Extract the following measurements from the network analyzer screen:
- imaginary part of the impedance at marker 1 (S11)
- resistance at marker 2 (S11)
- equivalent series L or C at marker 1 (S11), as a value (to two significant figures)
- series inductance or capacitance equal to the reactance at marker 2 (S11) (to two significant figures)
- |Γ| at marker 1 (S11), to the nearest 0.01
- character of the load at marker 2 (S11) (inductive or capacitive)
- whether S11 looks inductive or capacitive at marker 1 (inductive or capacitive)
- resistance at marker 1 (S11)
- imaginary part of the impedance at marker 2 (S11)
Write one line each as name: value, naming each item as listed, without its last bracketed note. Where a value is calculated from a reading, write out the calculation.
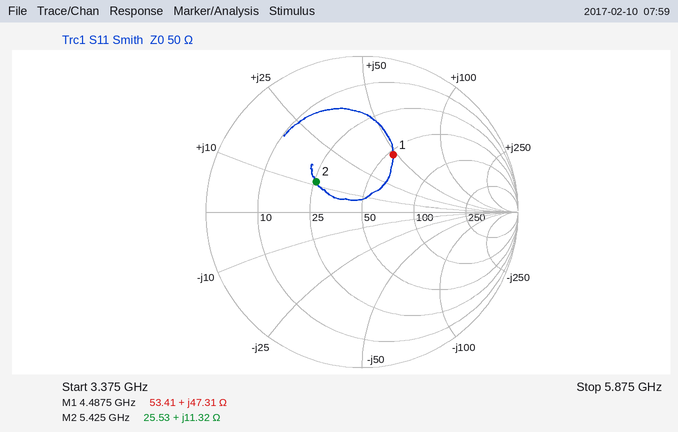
imaginary part of the impedance at marker 1: +47.31 Ω
resistance at marker 2: 25.53 Ω
equivalent series L or C at marker 1 (S11), as a value: L = 47.31 Ω/(2π × 4.4875 GHz) ≈ 1.7 nH
series inductance or capacitance equal to the reactance at marker 2 (S11): L = 11.32 Ω/(2π × 5.425 GHz) ≈ 332 pH, so 330 pH to two significant figures
|Γ| at marker 1 (S11), to the nearest 0.01: 0.42
character of the load at marker 2 (S11): inductive
whether S11 looks inductive or capacitive at marker 1: inductive
resistance at marker 1: 53.41 Ω
imaginary part of the impedance at marker 2: +11.32 Ω
